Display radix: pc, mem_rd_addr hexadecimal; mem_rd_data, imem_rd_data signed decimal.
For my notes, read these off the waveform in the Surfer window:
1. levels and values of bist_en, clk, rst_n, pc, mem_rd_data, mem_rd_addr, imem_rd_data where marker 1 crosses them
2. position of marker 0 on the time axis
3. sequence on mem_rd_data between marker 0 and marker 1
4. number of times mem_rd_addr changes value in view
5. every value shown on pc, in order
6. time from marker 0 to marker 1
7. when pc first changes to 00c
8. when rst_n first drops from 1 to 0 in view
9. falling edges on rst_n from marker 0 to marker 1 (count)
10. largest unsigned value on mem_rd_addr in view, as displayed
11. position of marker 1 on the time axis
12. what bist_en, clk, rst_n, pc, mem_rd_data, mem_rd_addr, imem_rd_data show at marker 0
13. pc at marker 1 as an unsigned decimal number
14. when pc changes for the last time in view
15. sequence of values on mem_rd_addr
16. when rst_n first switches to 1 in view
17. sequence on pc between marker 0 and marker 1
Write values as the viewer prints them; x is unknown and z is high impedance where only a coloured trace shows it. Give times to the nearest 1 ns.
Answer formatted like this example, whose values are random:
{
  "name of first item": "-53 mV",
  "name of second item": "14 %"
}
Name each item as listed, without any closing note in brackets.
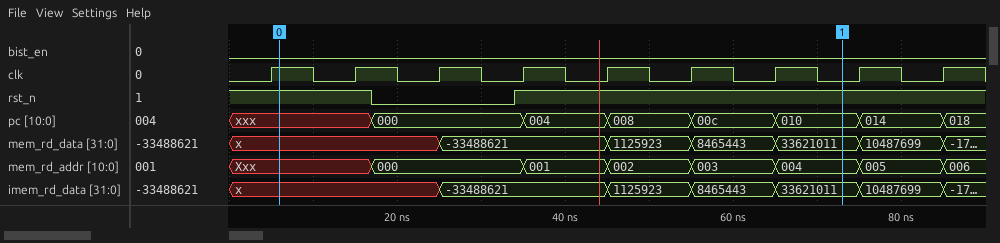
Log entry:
{
  "levels and values of bist_en, clk, rst_n, pc, mem_rd_data, mem_rd_addr, imem_rd_data where marker 1 crosses them": "bist_en=0, clk=0, rst_n=1, pc=010, mem_rd_data=33621011, mem_rd_addr=004, imem_rd_data=33621011",
  "position of marker 0 on the time axis": "6 ns",
  "sequence on mem_rd_data between marker 0 and marker 1": "x, -33488621, 1125923, 8465443, 33621011",
  "number of times mem_rd_addr changes value in view": "7",
  "every value shown on pc, in order": "xxx, 000, 004, 008, 00c, 010, 014, 018",
  "time from marker 0 to marker 1": "67 ns",
  "when pc first changes to 00c": "55 ns",
  "when rst_n first drops from 1 to 0 in view": "17 ns",
  "falling edges on rst_n from marker 0 to marker 1": "1",
  "largest unsigned value on mem_rd_addr in view, as displayed": "006",
  "position of marker 1 on the time axis": "73 ns",
  "what bist_en, clk, rst_n, pc, mem_rd_data, mem_rd_addr, imem_rd_data show at marker 0": "bist_en=0, clk=1, rst_n=1, pc=xxx, mem_rd_data=x, mem_rd_addr=Xxx, imem_rd_data=x",
  "pc at marker 1 as an unsigned decimal number": "16",
  "when pc changes for the last time in view": "85 ns",
  "sequence of values on mem_rd_addr": "Xxx, 000, 001, 002, 003, 004, 005, 006",
  "when rst_n first switches to 1 in view": "34 ns",
  "sequence on pc between marker 0 and marker 1": "xxx, 000, 004, 008, 00c, 010"
}
